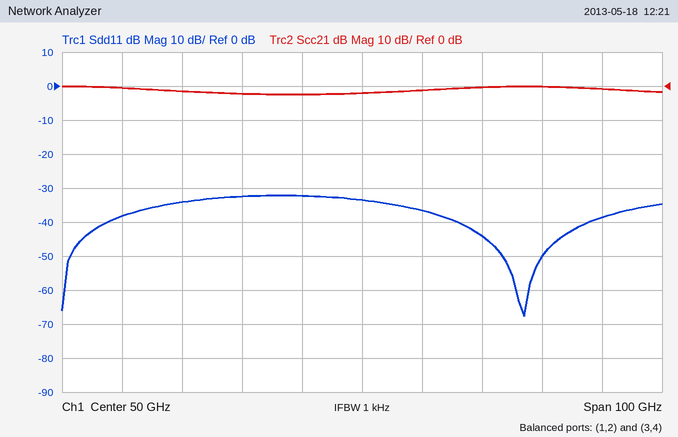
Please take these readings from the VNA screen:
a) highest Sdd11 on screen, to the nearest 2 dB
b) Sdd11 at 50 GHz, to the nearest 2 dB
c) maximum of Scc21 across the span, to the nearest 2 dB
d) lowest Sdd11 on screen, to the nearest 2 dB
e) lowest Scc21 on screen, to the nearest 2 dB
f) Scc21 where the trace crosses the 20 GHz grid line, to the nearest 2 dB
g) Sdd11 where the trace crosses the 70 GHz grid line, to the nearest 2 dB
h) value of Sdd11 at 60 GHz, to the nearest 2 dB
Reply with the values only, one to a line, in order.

-32 dB
-34 dB
0 dB
-68 dB
-2 dB
-2 dB
-44 dB
-36 dB
